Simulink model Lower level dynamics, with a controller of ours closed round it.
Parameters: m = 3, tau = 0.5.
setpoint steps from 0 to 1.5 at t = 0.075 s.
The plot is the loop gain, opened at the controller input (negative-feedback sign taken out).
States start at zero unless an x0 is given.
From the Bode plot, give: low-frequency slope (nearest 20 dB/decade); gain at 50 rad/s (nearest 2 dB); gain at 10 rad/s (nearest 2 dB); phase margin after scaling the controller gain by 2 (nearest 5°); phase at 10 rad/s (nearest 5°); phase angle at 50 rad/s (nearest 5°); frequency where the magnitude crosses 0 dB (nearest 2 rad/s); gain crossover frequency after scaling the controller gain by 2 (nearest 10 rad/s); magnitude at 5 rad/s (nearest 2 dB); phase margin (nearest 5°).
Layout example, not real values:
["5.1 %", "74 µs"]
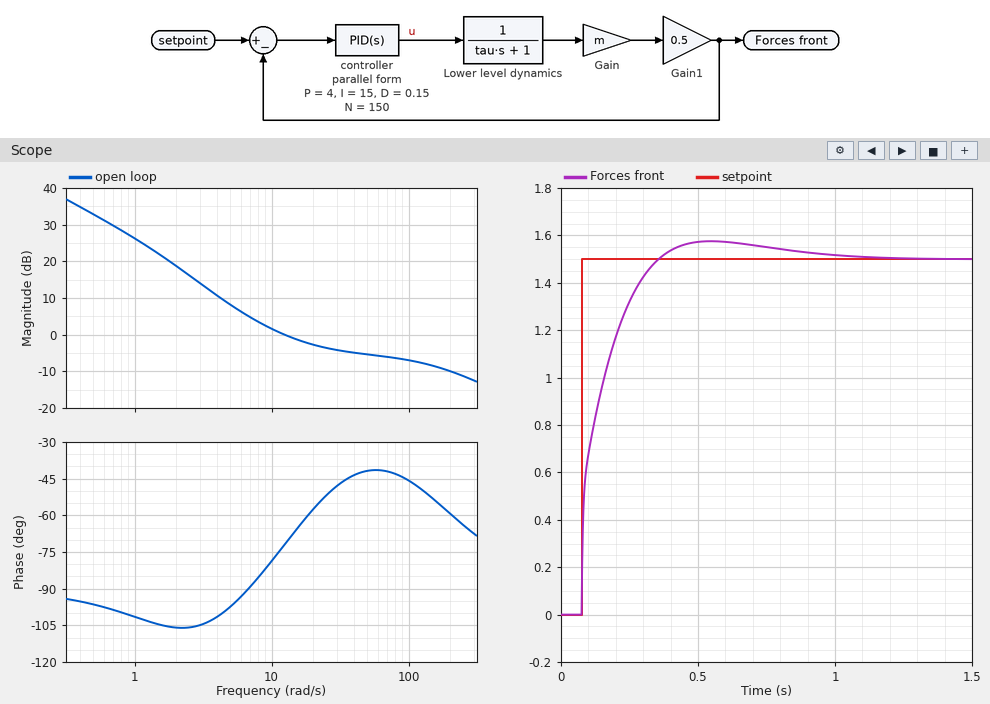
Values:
["-20 dB/decade", "-6 dB", "2 dB", "140°", "-80°", "-40°", "12 rad/s", "70 rad/s", "8 dB", "110°"]
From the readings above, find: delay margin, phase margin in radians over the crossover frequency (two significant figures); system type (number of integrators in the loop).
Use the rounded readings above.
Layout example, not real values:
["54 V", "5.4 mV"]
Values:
["0.16 s", "1"]
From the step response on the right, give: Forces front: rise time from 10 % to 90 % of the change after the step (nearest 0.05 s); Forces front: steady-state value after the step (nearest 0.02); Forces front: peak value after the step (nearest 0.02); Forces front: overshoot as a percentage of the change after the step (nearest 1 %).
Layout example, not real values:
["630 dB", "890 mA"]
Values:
["0.20 s", "1.50", "1.58", "5 %"]
